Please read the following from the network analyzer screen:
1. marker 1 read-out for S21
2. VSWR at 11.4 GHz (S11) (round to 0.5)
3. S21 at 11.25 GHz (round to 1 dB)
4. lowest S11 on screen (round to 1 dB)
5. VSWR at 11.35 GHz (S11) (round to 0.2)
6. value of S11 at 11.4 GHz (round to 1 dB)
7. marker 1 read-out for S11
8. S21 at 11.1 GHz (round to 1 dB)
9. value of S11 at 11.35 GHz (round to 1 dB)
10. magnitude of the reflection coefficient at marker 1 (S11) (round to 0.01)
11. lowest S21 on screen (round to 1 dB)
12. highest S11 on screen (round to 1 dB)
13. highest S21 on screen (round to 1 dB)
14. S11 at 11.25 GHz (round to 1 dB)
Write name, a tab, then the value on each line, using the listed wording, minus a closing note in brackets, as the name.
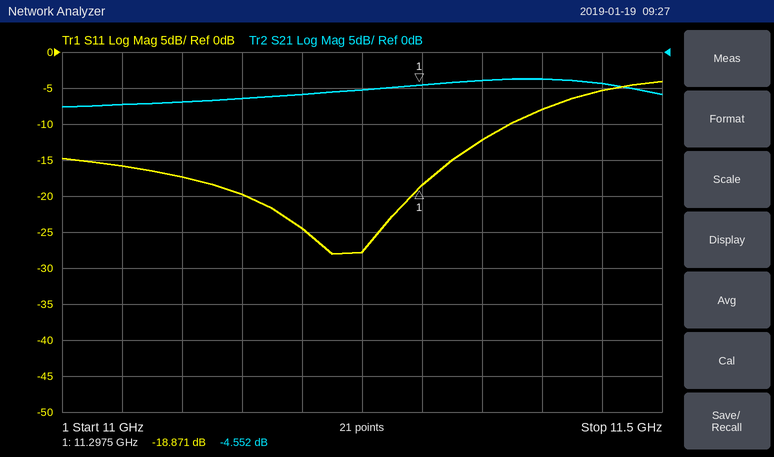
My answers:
marker 1 read-out for S21	-4.552 dB
VSWR at 11.4 GHz (S11)	2.5
S21 at 11.25 GHz	-5 dB
lowest S11 on screen	-28 dB
VSWR at 11.35 GHz (S11)	1.6
value of S11 at 11.4 GHz	-8 dB
marker 1 read-out for S11	-18.871 dB
S21 at 11.1 GHz	-7 dB
value of S11 at 11.35 GHz	-12 dB
magnitude of the reflection coefficient at marker 1 (S11)	0.11
lowest S21 on screen	-8 dB
highest S11 on screen	-4 dB
highest S21 on screen	-4 dB
S11 at 11.25 GHz	-28 dB
